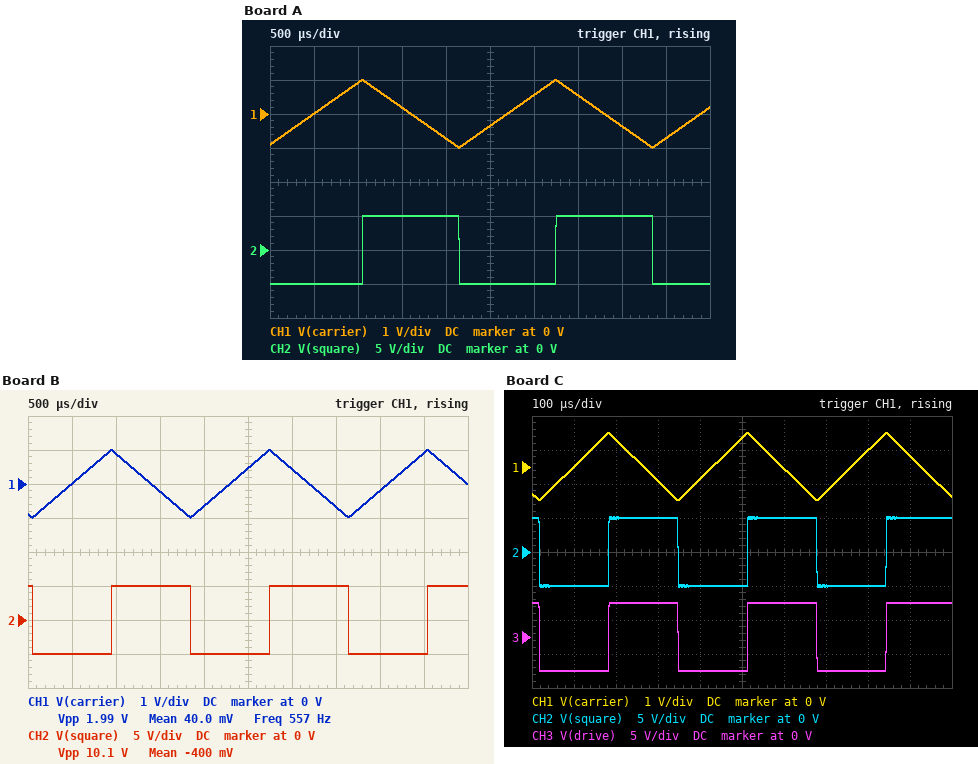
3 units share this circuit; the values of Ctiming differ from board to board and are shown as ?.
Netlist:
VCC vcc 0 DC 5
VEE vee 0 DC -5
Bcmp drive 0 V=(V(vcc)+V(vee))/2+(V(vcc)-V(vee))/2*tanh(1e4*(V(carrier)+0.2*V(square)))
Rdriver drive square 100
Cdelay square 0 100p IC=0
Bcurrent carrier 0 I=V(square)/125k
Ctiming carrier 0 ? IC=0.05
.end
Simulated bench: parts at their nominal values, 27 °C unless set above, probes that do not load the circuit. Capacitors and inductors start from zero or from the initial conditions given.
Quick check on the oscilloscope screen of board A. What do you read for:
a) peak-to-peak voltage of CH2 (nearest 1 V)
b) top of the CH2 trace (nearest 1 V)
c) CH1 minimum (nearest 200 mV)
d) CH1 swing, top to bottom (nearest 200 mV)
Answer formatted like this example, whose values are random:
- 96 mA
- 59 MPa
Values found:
- 10 V
- 5 V
- -1.0 V
- 2.0 V
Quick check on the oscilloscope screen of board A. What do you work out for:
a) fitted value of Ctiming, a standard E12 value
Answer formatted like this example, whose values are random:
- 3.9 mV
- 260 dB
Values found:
- 22 nF
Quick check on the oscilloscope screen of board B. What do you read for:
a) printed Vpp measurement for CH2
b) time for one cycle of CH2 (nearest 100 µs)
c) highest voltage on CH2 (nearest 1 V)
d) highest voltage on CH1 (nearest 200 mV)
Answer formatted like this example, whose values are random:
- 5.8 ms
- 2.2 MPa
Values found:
- 10.1 V
- 1.8 ms
- 5 V
- 1.0 V
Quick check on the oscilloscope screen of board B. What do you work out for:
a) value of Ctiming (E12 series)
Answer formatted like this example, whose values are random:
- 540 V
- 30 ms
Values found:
- 18 nF
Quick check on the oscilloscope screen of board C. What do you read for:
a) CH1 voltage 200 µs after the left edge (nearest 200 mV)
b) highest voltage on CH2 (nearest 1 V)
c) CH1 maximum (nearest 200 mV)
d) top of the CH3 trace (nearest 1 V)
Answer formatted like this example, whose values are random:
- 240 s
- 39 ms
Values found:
- 800 mV
- 5 V
- 1.0 V
- 5 V
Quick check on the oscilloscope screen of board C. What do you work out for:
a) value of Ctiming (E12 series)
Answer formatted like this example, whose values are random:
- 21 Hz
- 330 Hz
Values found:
- 3.3 nF
